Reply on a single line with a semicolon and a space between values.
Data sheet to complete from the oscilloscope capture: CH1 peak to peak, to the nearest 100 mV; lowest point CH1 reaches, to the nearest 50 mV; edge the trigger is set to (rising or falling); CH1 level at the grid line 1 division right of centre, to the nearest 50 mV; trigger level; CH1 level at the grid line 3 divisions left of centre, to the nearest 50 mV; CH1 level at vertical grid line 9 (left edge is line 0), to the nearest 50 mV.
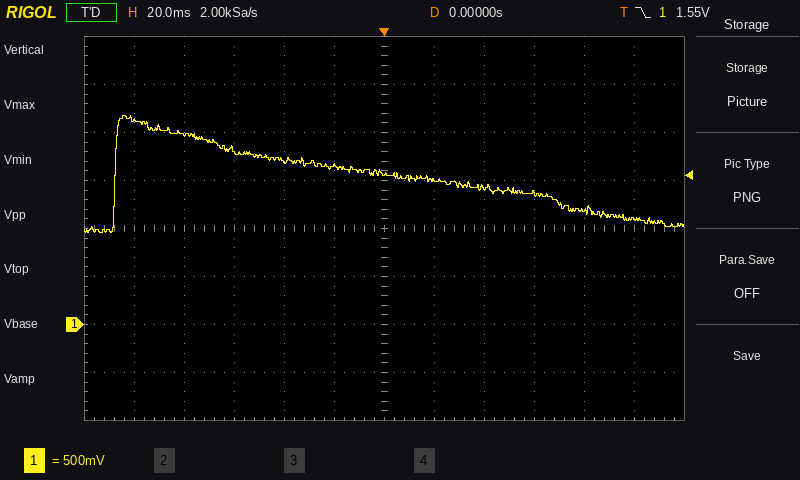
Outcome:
1.20 V; 950 mV; falling; 1.50 V; 1.55 V; 1.80 V; 1.35 V
